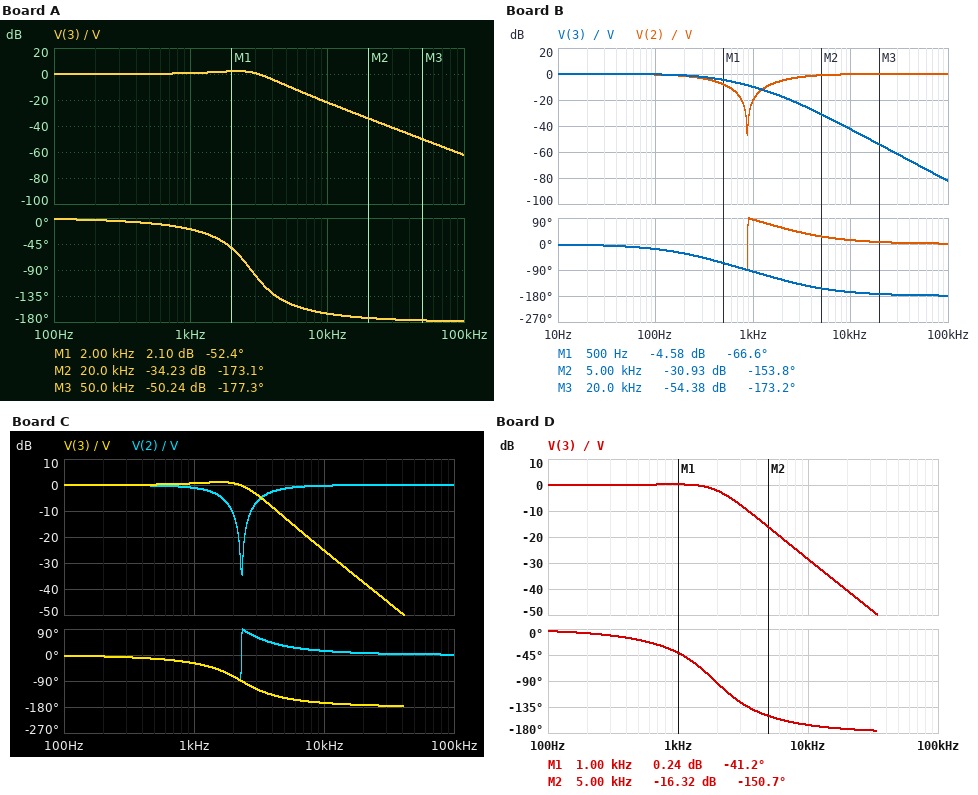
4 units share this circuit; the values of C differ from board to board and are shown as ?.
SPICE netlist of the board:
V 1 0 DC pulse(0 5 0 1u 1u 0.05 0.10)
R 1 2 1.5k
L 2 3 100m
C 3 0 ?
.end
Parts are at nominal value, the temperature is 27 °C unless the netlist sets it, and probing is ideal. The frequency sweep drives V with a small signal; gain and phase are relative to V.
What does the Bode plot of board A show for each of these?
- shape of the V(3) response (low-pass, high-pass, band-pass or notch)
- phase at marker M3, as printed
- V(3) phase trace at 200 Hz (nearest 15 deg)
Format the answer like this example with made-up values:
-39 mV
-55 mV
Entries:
low-pass
-177.3 deg
0 deg
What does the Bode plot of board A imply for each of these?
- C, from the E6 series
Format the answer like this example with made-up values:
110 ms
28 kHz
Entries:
33 nF
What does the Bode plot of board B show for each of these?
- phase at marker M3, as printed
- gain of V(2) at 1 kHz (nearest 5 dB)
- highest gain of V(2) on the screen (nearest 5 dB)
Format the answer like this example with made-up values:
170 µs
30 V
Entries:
-173.2 deg
-20 dB
0 dB
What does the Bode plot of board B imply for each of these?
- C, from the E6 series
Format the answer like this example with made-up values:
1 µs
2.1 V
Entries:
330 nF
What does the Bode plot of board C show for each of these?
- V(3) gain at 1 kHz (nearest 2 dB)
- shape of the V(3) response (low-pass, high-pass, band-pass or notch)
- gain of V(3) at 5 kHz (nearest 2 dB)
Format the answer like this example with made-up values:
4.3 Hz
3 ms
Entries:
0 dB
low-pass
-12 dB
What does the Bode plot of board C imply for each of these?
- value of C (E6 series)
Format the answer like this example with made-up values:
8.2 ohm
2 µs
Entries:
47 nF
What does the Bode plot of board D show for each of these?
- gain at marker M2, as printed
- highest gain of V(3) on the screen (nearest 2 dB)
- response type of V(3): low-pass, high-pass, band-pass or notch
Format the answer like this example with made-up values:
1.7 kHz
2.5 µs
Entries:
-16.32 dB
0 dB
low-pass
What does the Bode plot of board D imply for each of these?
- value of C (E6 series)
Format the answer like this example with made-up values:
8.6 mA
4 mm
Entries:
68 nF
